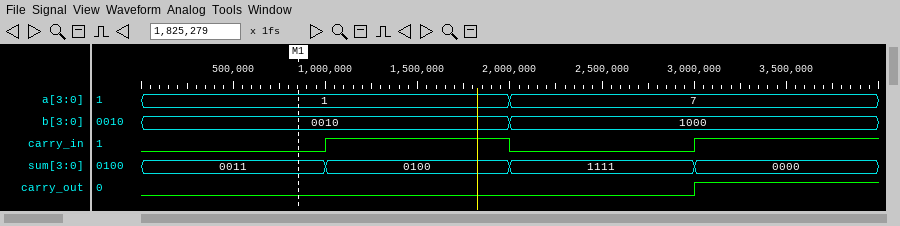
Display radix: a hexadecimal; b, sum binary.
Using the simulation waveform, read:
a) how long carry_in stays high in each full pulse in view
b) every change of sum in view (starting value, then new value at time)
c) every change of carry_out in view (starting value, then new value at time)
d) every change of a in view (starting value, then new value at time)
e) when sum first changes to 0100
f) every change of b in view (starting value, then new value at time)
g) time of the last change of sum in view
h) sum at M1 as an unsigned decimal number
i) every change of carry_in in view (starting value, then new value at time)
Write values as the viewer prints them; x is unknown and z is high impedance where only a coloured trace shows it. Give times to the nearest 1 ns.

1 ns
0011, 0100 at 1 ns, 1111 at 2 ns, 0000 at 3 ns
0, 1 at 3 ns
1, 7 at 2 ns
1 ns
0010, 1000 at 2 ns
3 ns
3
0, 1 at 1 ns, 0 at 2 ns, 1 at 3 ns
